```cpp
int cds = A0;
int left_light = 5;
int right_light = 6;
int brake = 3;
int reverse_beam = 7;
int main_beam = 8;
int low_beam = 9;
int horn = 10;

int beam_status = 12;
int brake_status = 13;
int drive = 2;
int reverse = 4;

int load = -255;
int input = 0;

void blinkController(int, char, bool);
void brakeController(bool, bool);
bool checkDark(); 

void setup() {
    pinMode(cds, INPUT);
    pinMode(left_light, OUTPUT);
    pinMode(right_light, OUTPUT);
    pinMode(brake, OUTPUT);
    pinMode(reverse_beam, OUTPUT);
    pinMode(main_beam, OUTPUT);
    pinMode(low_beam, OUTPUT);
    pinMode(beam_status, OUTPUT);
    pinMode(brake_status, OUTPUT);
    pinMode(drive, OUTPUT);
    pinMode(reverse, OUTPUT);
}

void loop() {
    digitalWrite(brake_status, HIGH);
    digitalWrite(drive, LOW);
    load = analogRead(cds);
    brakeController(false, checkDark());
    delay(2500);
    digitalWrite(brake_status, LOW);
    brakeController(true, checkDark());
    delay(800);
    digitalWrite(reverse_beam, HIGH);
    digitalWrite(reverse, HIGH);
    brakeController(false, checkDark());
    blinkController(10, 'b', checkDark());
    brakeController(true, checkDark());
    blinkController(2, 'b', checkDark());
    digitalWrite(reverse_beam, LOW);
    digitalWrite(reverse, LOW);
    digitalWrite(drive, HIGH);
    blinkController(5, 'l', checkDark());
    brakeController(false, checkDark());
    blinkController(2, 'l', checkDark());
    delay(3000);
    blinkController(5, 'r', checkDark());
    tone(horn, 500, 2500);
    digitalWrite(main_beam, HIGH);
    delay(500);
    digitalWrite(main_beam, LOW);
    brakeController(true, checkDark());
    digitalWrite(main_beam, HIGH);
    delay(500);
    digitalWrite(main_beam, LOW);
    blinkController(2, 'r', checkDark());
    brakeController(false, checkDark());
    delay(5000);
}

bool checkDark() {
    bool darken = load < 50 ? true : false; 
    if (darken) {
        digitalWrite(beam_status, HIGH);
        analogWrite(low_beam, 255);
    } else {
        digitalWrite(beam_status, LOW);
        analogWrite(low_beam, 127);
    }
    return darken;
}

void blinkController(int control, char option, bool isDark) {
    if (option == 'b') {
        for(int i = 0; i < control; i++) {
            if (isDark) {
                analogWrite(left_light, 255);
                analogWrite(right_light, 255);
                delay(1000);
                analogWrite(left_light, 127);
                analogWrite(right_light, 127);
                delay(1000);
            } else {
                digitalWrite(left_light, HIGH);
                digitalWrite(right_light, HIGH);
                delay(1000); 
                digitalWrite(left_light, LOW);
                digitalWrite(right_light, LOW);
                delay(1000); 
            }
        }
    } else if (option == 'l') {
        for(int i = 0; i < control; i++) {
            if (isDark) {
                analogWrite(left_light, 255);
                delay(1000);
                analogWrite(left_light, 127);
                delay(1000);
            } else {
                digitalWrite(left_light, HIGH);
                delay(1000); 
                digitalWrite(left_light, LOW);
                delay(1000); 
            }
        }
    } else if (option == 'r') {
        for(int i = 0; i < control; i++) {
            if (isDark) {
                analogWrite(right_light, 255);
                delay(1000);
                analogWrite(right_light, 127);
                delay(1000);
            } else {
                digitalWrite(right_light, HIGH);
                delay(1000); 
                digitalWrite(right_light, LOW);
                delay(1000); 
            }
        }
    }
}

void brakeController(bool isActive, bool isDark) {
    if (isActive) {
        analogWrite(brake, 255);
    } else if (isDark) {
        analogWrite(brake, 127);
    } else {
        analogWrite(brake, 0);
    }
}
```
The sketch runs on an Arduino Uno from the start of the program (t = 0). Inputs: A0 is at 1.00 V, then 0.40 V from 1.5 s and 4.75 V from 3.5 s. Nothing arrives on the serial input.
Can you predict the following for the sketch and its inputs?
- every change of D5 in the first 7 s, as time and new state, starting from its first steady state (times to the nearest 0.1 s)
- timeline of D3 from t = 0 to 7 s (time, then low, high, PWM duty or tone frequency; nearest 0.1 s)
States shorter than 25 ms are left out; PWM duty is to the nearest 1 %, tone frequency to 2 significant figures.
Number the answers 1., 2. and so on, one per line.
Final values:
1. 0 s low; 3.3 s high; 4.3 s low; 5.3 s high; 6.3 s low
2. 0 s low; 2.5 s high; 3.3 s low
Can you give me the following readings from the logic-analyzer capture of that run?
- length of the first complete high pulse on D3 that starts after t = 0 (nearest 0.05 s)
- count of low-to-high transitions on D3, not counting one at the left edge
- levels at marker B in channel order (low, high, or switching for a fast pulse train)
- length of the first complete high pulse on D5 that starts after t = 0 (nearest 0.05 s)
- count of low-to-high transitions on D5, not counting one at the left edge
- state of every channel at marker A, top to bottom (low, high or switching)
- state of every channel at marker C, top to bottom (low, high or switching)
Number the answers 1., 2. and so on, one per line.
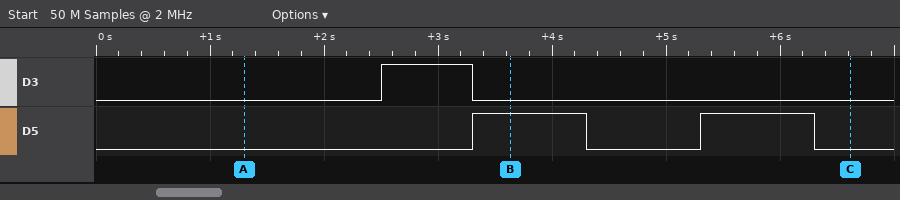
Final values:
1. 0.80 s
2. 1
3. D3 low, D5 high
4. 1.00 s
5. 2
6. D3 low, D5 low
7. D3 low, D5 low
